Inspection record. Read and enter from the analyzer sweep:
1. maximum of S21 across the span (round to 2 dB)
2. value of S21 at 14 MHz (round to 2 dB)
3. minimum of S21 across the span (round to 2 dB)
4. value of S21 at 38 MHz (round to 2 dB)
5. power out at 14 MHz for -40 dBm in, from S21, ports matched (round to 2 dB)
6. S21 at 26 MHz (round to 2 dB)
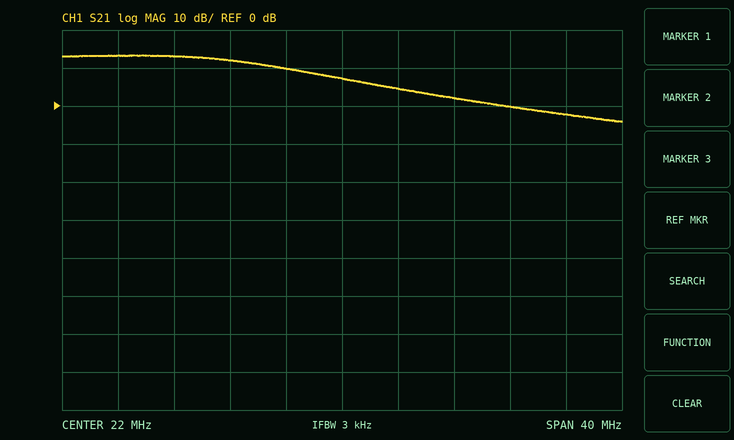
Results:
14 dB
12 dB
-4 dB
-2 dB
-28 dBm
4 dB
